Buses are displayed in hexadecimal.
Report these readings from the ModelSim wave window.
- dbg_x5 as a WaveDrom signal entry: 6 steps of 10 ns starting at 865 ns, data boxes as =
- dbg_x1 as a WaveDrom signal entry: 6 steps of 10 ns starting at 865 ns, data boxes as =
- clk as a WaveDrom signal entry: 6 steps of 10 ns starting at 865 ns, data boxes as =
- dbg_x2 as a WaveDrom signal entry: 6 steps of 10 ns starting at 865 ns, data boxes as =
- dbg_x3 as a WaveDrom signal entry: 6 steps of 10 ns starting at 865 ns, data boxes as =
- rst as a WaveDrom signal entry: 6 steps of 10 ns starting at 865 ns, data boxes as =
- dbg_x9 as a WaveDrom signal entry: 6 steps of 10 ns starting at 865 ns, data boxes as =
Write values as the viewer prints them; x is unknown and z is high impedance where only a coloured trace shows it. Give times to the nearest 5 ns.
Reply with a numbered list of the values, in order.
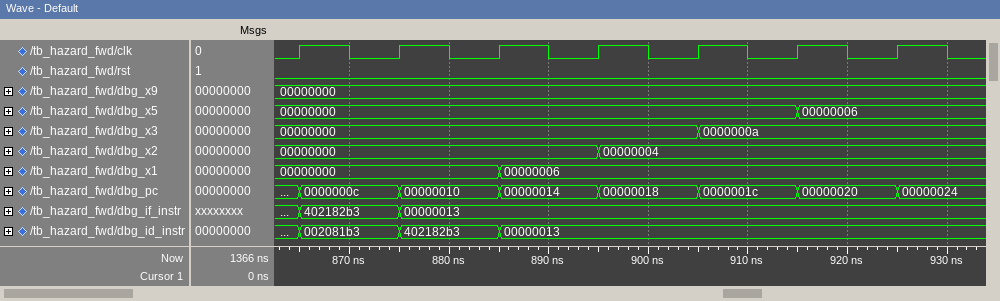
1. {name: 'dbg_x5', wave: '=....=', data: '00000000 00000006'}
2. {name: 'dbg_x1', wave: '=.=...', data: '00000000 00000006'}
3. {name: 'clk', wave: 'p.....'}
4. {name: 'dbg_x2', wave: '=..=..', data: '00000000 00000004'}
5. {name: 'dbg_x3', wave: '=...=.', data: '00000000 0000000a'}
6. {name: 'rst', wave: '0.....'}
7. {name: 'dbg_x9', wave: '=.....', data: '00000000'}
